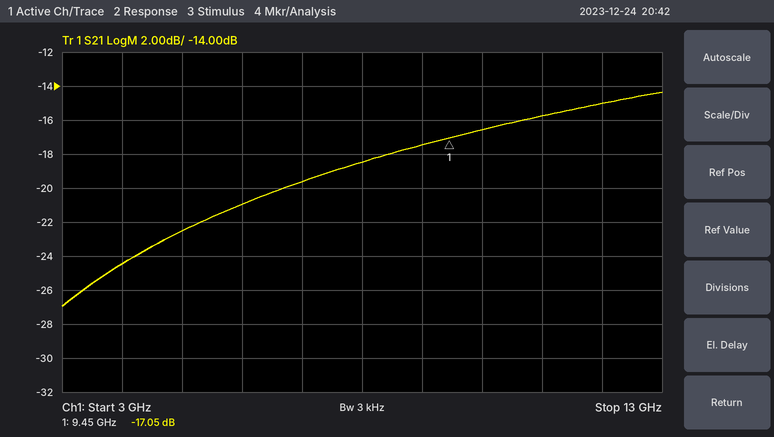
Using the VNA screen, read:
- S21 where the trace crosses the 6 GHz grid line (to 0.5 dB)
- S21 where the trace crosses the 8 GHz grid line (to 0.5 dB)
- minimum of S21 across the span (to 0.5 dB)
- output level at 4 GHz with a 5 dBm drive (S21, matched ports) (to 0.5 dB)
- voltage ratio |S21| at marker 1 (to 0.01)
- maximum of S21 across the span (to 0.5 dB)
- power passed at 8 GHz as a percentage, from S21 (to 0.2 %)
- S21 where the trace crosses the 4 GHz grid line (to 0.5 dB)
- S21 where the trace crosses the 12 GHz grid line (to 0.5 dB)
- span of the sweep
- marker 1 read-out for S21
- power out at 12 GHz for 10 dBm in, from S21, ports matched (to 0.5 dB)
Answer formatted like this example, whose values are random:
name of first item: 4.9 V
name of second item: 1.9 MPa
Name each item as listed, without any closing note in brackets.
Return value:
S21 where the trace crosses the 6 GHz grid line: -21.0 dB
S21 where the trace crosses the 8 GHz grid line: -18.5 dB
minimum of S21 across the span: -27.0 dB
output level at 4 GHz with a 5 dBm drive (S21, matched ports): -19.5 dBm
voltage ratio |S21| at marker 1: 0.14
maximum of S21 across the span: -14.5 dB
power passed at 8 GHz as a percentage, from S21: 1.4 %
S21 where the trace crosses the 4 GHz grid line: -24.5 dB
S21 where the trace crosses the 12 GHz grid line: -15.0 dB
span of the sweep: 10 GHz
marker 1 read-out for S21: -17.05 dB
power out at 12 GHz for 10 dBm in, from S21, ports matched: -5.0 dBm
